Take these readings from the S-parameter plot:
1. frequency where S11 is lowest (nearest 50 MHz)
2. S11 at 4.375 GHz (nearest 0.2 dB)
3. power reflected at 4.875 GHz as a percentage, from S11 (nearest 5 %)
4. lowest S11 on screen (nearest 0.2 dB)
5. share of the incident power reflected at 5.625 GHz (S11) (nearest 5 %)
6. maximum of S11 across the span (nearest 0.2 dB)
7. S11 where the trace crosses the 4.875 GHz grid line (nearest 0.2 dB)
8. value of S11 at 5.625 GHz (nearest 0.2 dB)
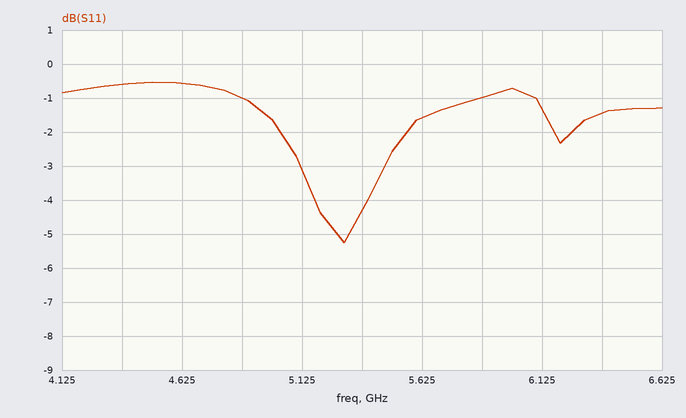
5.30 GHz
-0.6 dB
80 %
-5.2 dB
70 %
-0.6 dB
-1.0 dB
-1.6 dB
